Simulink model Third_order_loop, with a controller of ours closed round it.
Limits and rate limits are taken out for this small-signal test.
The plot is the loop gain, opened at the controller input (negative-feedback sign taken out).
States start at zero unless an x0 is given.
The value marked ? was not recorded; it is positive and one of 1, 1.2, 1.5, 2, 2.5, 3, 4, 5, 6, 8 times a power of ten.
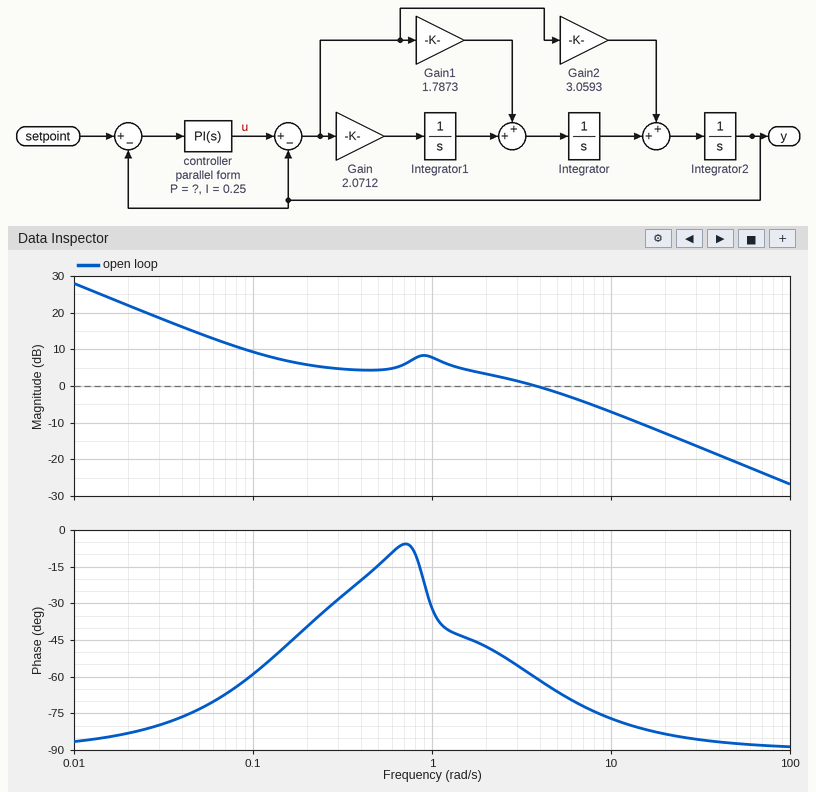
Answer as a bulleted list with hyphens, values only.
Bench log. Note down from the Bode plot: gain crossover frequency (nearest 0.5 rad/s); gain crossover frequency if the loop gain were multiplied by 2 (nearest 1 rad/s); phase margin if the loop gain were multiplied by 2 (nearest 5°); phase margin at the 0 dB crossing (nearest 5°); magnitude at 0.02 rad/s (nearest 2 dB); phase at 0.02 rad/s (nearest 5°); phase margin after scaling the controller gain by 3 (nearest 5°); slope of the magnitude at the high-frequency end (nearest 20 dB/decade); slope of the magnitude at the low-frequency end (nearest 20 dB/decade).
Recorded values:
- 4.0 rad/s
- 9 rad/s
- 105°
- 120°
- 22 dB
- -85°
- 100°
- -20 dB/decade
- -20 dB/decade
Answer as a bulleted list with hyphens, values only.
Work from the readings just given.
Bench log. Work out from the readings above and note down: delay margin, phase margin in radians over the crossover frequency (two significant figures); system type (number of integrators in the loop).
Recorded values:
- 0.52 s
- 1
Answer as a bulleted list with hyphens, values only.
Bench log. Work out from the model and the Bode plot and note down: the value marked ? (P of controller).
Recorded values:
- 1.5
